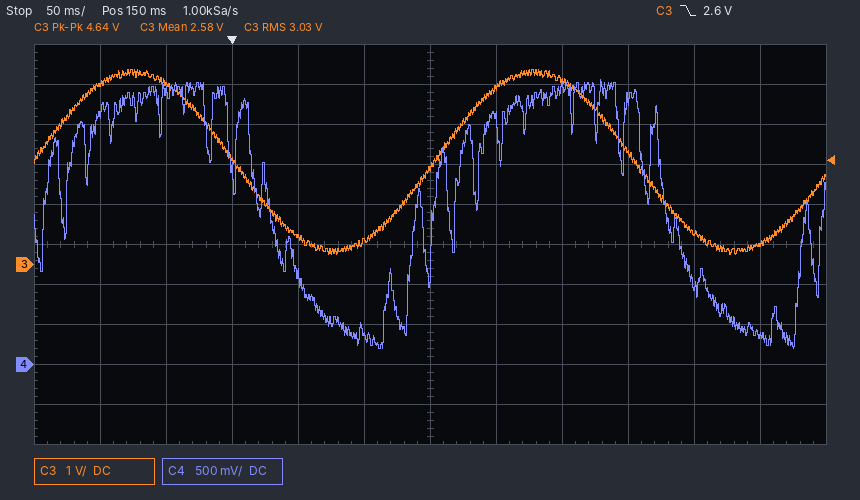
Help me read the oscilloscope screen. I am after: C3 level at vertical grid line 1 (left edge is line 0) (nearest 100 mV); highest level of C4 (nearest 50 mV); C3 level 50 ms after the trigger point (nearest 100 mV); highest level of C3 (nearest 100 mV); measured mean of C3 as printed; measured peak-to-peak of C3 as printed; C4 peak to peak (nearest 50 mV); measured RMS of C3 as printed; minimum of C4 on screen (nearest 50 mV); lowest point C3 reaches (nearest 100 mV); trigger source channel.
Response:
4.5 V
3.55 V
700 mV
4.9 V
2.58 V
4.64 V
3.35 V
3.03 V
200 mV
200 mV
C3
